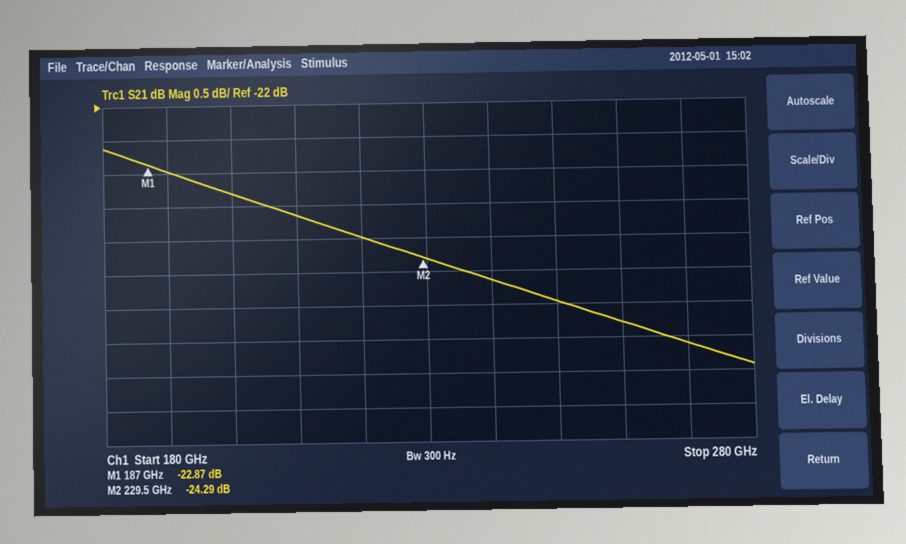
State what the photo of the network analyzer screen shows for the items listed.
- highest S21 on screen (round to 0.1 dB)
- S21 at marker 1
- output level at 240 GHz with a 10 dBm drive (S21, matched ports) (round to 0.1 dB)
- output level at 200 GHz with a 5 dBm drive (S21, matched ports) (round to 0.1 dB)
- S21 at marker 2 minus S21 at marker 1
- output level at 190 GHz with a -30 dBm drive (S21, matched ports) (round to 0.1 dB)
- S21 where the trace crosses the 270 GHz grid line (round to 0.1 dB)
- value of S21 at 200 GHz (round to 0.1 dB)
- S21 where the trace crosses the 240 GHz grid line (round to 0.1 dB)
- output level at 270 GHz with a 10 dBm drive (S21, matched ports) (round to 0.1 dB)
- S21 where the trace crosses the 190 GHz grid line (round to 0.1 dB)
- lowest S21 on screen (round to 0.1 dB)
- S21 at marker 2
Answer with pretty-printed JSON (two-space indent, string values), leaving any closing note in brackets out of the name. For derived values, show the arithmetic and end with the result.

{
  "highest S21 on screen": "-22.6 dB",
  "S21 at marker 1": "-22.87 dB",
  "output level at 240 GHz with a 10 dBm drive (S21, matched ports)": "10 dBm + (-24.6 dB) = -14.6 dBm",
  "output level at 200 GHz with a 5 dBm drive (S21, matched ports)": "5 dBm + (-23.3 dB) = -18.3 dBm",
  "S21 at marker 2 minus S21 at marker 1": "-24.29 − (-22.87) = -1.42 dB",
  "output level at 190 GHz with a -30 dBm drive (S21, matched ports)": "-30 dBm + (-23.0 dB) = -53.0 dBm",
  "S21 where the trace crosses the 270 GHz grid line": "-25.6 dB",
  "value of S21 at 200 GHz": "-23.3 dB",
  "S21 where the trace crosses the 240 GHz grid line": "-24.6 dB",
  "output level at 270 GHz with a 10 dBm drive (S21, matched ports)": "10 dBm + (-25.6 dB) = -15.6 dBm",
  "S21 where the trace crosses the 190 GHz grid line": "-23.0 dB",
  "lowest S21 on screen": "-25.9 dB",
  "S21 at marker 2": "-24.29 dB"
}
